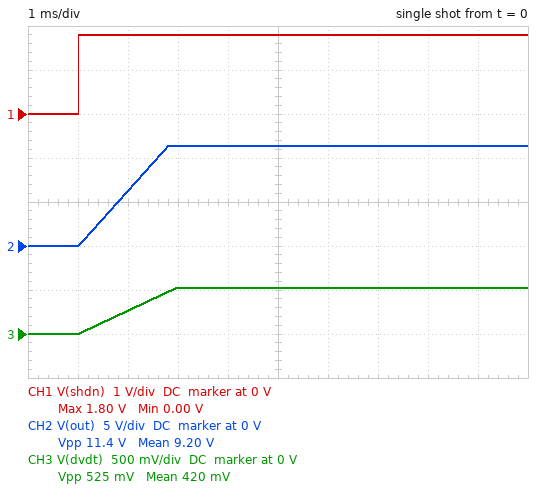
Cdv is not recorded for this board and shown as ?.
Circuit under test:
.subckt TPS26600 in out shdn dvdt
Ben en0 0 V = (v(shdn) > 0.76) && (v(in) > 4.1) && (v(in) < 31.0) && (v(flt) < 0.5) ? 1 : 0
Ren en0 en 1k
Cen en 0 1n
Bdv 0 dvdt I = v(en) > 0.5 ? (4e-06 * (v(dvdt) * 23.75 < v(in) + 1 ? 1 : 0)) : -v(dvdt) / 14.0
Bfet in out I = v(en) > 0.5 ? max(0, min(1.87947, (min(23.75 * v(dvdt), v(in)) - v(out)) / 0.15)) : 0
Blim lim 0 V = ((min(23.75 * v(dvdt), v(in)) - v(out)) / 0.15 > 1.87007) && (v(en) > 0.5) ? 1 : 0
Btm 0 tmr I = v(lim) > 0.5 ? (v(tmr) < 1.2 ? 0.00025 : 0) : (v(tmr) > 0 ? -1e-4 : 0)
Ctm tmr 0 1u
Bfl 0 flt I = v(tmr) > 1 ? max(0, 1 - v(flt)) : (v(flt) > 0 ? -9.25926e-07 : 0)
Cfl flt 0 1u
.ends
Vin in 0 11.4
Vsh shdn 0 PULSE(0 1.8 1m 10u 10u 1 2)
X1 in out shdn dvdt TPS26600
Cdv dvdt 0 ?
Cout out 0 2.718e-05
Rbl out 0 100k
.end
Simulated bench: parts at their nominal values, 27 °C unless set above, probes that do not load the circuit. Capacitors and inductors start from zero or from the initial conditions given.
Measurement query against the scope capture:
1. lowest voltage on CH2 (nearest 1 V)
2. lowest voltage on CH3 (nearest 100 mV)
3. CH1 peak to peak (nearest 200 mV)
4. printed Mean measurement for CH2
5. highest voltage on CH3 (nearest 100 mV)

0 V
0 V
1.8 V
9.20 V
500 mV
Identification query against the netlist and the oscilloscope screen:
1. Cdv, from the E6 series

15 nF
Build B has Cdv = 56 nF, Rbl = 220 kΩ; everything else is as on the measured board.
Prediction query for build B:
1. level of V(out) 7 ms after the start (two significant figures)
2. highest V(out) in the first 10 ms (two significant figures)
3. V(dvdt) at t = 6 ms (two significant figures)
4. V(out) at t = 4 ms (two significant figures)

10 V
11 V
360 mV
5.1 V
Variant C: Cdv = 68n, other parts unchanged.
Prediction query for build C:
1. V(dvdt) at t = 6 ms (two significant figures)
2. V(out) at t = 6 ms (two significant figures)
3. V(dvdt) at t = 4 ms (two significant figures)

290 mV
7.0 V
180 mV
